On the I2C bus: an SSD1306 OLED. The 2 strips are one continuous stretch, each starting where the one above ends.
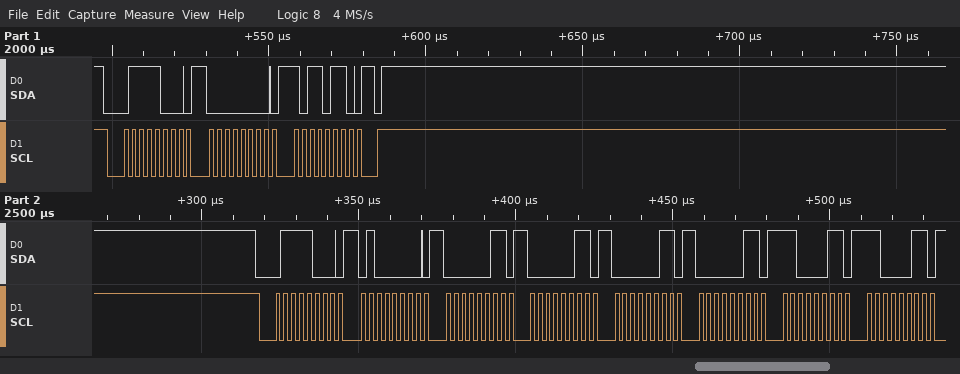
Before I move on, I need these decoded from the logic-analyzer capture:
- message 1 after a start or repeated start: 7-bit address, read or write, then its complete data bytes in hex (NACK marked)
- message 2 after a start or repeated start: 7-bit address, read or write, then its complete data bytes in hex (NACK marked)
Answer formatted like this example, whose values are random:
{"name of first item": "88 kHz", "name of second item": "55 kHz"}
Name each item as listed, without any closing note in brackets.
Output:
{"message 1 after a start or repeated start: 7-bit address, read or write, then its complete data bytes in hex": "0x3C write: 00 B6", "message 2 after a start or repeated start: 7-bit address, read or write, then its complete data bytes in hex": "0x3C write: 40 03 03 03 03 C3 C3"}
